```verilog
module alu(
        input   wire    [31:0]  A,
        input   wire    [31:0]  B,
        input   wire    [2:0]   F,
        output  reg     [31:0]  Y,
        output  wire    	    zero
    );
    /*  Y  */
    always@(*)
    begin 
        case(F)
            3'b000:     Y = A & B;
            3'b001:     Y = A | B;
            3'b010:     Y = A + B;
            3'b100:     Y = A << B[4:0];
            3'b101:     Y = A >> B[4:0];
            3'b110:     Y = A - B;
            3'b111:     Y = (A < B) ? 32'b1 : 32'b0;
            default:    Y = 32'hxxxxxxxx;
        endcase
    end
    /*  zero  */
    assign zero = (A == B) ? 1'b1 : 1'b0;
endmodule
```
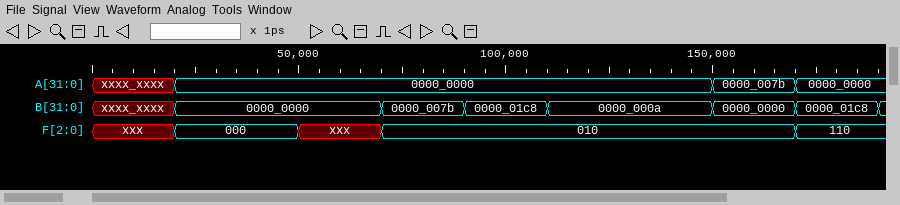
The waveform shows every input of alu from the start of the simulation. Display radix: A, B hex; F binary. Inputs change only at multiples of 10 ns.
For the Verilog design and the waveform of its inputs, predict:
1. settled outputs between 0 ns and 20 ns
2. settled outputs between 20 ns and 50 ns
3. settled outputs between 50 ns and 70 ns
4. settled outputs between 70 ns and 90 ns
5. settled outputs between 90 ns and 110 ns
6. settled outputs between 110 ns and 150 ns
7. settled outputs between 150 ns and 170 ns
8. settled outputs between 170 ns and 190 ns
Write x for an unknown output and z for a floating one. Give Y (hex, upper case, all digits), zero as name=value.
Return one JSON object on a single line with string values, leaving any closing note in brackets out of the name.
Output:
{"settled outputs between 0 ns and 20 ns": "Y=x, zero=x", "settled outputs between 20 ns and 50 ns": "Y=00000000, zero=1", "settled outputs between 50 ns and 70 ns": "Y=x, zero=1", "settled outputs between 70 ns and 90 ns": "Y=0000007B, zero=0", "settled outputs between 90 ns and 110 ns": "Y=000001C8, zero=0", "settled outputs between 110 ns and 150 ns": "Y=0000000A, zero=0", "settled outputs between 150 ns and 170 ns": "Y=0000007B, zero=0", "settled outputs between 170 ns and 190 ns": "Y=FFFFFE38, zero=0"}
